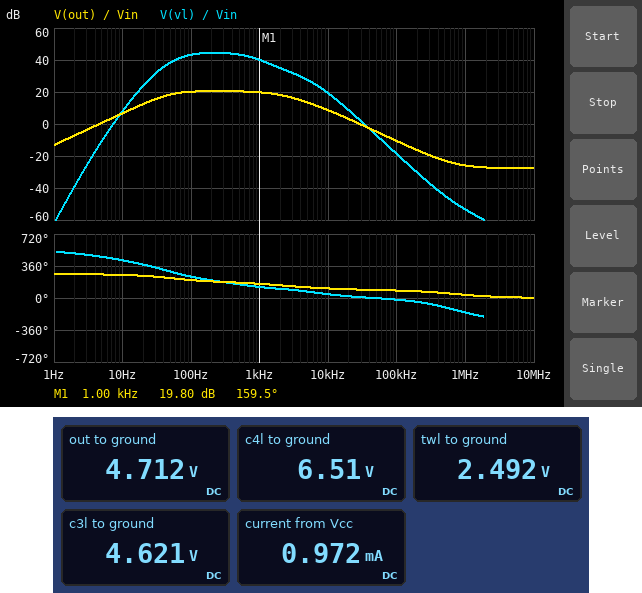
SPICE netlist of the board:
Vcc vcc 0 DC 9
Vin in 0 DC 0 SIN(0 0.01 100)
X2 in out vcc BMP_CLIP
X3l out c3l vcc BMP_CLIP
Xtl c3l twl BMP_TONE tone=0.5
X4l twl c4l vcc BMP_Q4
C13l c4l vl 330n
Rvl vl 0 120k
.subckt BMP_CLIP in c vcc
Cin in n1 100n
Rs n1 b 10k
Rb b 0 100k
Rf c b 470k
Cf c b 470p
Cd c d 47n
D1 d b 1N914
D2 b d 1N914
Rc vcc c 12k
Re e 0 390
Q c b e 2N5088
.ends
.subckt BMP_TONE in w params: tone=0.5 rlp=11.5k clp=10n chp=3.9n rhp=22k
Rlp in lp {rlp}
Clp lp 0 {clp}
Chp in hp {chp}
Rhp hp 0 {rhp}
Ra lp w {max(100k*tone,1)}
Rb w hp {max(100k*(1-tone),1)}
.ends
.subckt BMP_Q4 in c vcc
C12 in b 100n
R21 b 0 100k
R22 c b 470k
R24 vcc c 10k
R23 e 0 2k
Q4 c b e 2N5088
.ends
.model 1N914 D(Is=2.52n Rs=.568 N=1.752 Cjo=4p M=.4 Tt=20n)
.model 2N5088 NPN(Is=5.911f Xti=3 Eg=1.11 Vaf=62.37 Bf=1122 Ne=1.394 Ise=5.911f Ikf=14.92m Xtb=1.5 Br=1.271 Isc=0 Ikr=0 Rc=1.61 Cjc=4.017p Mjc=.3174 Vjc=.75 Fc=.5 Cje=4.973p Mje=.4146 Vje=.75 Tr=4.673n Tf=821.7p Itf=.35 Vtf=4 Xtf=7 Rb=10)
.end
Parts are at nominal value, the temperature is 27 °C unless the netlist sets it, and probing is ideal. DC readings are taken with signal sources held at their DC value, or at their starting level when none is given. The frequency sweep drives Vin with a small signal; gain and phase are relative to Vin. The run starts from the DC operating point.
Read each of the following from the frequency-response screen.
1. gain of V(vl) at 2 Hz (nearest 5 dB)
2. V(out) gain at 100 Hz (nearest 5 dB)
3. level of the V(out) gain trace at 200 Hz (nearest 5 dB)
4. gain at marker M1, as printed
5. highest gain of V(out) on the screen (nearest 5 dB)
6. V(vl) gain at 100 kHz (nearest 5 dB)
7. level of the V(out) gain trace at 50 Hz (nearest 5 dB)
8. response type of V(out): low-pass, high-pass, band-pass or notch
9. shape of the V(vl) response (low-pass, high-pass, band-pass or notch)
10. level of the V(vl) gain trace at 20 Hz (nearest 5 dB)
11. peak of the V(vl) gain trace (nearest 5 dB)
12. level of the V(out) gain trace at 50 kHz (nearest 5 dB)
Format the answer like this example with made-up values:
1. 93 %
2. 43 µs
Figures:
1. -40 dB
2. 20 dB
3. 20 dB
4. 19.80 dB
5. 20 dB
6. -20 dB
7. 20 dB
8. band-pass
9. band-pass
10. 25 dB
11. 45 dB
12. -5 dB
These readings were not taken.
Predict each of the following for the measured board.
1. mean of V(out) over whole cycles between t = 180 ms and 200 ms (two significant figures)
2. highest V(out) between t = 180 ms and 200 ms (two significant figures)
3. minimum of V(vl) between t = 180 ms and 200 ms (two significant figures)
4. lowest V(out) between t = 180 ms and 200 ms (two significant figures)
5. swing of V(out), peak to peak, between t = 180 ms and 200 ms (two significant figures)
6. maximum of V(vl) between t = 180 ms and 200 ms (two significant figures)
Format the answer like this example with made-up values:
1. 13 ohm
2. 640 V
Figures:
1. 4.7 V
2. 4.8 V
3. -450 mV
4. 4.6 V
5. 200 mV
6. 450 mV
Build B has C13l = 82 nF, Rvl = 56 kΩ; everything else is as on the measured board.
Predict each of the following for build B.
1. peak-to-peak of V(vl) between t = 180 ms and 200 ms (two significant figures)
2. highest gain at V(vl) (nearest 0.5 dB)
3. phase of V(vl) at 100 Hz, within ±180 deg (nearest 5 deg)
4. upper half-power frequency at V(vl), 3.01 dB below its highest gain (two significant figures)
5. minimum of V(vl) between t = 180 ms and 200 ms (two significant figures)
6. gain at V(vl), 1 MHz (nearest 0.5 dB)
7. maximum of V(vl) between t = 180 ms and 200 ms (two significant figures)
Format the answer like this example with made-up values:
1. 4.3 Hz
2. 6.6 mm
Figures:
1. 820 mV
2. 44.0 dB
3. -105 deg
4. 800 Hz
5. -410 mV
6. -54.0 dB
7. 410 mV
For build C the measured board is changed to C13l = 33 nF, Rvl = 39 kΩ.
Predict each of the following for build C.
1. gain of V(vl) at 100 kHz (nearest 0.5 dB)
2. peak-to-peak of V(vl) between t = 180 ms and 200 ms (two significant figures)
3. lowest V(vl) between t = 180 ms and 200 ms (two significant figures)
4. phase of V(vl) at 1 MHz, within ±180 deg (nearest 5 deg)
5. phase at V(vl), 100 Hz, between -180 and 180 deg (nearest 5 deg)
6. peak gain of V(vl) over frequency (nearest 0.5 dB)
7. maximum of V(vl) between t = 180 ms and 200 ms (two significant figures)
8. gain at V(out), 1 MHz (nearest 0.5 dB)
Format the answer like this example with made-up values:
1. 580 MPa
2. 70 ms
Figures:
1. -20.0 dB
2. 820 mV
3. -410 mV
4. -160 deg
5. -75 deg
6. 43.0 dB
7. 410 mV
8. -26.0 dB
